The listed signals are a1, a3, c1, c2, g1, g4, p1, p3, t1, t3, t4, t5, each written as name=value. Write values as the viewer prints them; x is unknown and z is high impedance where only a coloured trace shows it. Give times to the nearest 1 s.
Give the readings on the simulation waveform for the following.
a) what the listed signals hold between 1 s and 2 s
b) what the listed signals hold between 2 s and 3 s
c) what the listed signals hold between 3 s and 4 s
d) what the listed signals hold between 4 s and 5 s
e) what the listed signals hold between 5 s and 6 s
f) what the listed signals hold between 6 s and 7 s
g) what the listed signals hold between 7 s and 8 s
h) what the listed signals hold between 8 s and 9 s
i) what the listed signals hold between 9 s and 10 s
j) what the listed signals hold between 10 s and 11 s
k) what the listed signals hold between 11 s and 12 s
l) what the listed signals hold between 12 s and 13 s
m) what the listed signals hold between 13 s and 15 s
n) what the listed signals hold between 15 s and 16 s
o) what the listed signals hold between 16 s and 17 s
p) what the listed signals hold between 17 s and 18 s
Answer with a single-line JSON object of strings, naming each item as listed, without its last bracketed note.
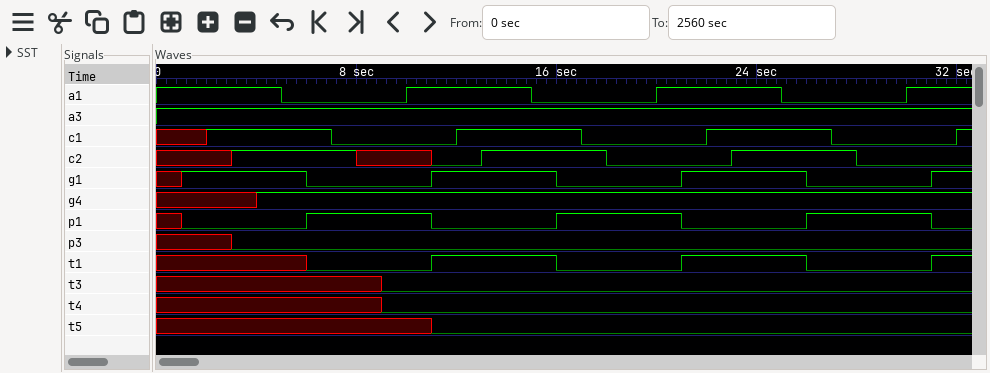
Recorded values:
{"what the listed signals hold between 1 s and 2 s": "a1=1, a3=1, c1=x, c2=x, g1=1, g4=x, p1=0, p3=x, t1=x, t3=x, t4=x, t5=x", "what the listed signals hold between 2 s and 3 s": "a1=1, a3=1, c1=1, c2=x, g1=1, g4=x, p1=0, p3=x, t1=x, t3=x, t4=x, t5=x", "what the listed signals hold between 3 s and 4 s": "a1=1, a3=1, c1=1, c2=1, g1=1, g4=x, p1=0, p3=0, t1=x, t3=x, t4=x, t5=x", "what the listed signals hold between 4 s and 5 s": "a1=1, a3=1, c1=1, c2=1, g1=1, g4=1, p1=0, p3=0, t1=x, t3=x, t4=x, t5=x", "what the listed signals hold between 5 s and 6 s": "a1=0, a3=1, c1=1, c2=1, g1=1, g4=1, p1=0, p3=0, t1=x, t3=x, t4=x, t5=x", "what the listed signals hold between 6 s and 7 s": "a1=0, a3=1, c1=1, c2=1, g1=0, g4=1, p1=1, p3=0, t1=0, t3=x, t4=x, t5=x", "what the listed signals hold between 7 s and 8 s": "a1=0, a3=1, c1=0, c2=1, g1=0, g4=1, p1=1, p3=0, t1=0, t3=x, t4=x, t5=x", "what the listed signals hold between 8 s and 9 s": "a1=0, a3=1, c1=0, c2=x, g1=0, g4=1, p1=1, p3=0, t1=0, t3=x, t4=x, t5=x", "what the listed signals hold between 9 s and 10 s": "a1=0, a3=1, c1=0, c2=x, g1=0, g4=1, p1=1, p3=0, t1=0, t3=0, t4=0, t5=x", "what the listed signals hold between 10 s and 11 s": "a1=1, a3=1, c1=0, c2=x, g1=0, g4=1, p1=1, p3=0, t1=0, t3=0, t4=0, t5=x", "what the listed signals hold between 11 s and 12 s": "a1=1, a3=1, c1=0, c2=0, g1=1, g4=1, p1=0, p3=0, t1=1, t3=0, t4=0, t5=0", "what the listed signals hold between 12 s and 13 s": "a1=1, a3=1, c1=1, c2=0, g1=1, g4=1, p1=0, p3=0, t1=1, t3=0, t4=0, t5=0", "what the listed signals hold between 13 s and 15 s": "a1=1, a3=1, c1=1, c2=1, g1=1, g4=1, p1=0, p3=0, t1=1, t3=0, t4=0, t5=0", "what the listed signals hold between 15 s and 16 s": "a1=0, a3=1, c1=1, c2=1, g1=1, g4=1, p1=0, p3=0, t1=1, t3=0, t4=0, t5=0", "what the listed signals hold between 16 s and 17 s": "a1=0, a3=1, c1=1, c2=1, g1=0, g4=1, p1=1, p3=0, t1=0, t3=0, t4=0, t5=0", "what the listed signals hold between 17 s and 18 s": "a1=0, a3=1, c1=0, c2=1, g1=0, g4=1, p1=1, p3=0, t1=0, t3=0, t4=0, t5=0"}
